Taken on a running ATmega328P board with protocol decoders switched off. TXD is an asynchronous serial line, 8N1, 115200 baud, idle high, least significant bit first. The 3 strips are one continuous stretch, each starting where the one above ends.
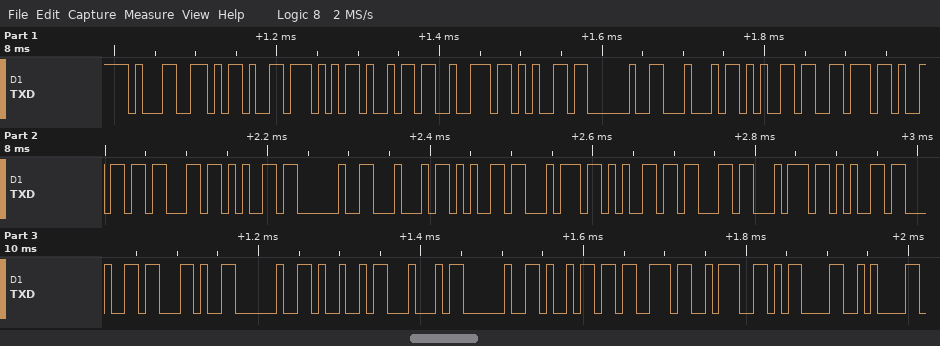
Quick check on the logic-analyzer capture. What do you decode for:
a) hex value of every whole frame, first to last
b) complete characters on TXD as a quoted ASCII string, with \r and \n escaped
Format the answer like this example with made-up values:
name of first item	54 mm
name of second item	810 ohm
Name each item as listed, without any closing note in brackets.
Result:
hex value of every whole frame, first to last	31 2D 57 69 72 65 20 44 65 76 69 63 65 20 44 65 74 65 63 74 65 64 2C 20 49 44 20 69 73 3A 0D 0A
complete characters on TXD as a quoted ASCII string, with \r and \n escaped	"1-Wire Device Detected, ID is:\r\n"
